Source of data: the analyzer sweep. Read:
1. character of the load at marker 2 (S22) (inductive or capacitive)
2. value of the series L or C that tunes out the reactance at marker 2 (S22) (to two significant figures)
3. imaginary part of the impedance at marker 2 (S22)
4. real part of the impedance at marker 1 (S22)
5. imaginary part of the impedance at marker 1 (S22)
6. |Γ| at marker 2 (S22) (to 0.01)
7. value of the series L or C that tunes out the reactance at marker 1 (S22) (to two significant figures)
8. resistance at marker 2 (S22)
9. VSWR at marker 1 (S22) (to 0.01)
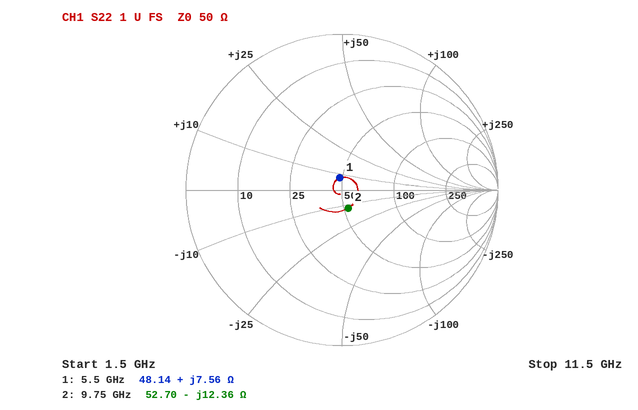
capacitive
200 pH
-12.36 Ω
48.14 Ω
+7.56 Ω
0.12
3.8 pF
52.70 Ω
1.17
